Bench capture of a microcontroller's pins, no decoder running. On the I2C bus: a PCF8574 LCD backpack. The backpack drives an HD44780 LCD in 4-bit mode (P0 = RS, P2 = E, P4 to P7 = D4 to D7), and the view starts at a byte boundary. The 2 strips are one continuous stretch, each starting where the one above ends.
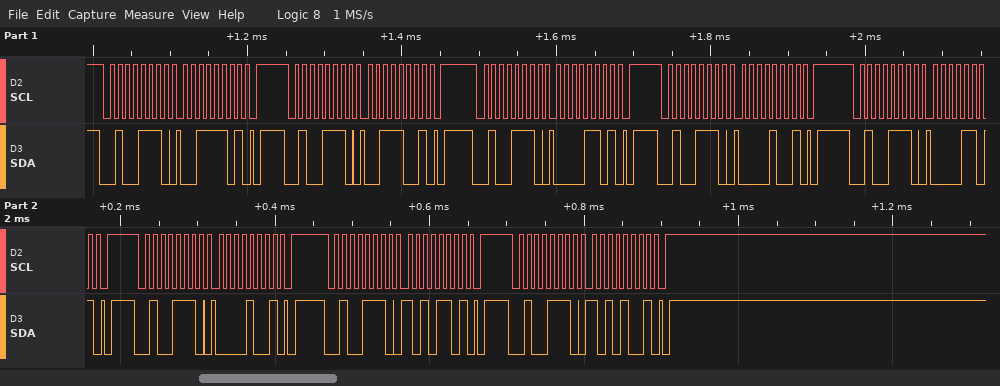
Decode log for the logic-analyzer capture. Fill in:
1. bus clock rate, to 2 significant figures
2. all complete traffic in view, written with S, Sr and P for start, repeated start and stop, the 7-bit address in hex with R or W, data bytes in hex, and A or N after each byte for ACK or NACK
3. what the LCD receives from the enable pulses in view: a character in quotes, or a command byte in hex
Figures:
100 kHz
S 27W A 3D A P S 27W A 39 A P S 27W A 0D A P S 27W A 09 A P S 27W A 0D A P S 27W A 09 A P S 27W A AD A P S 27W A A9 A P
'0' data 0x0A
